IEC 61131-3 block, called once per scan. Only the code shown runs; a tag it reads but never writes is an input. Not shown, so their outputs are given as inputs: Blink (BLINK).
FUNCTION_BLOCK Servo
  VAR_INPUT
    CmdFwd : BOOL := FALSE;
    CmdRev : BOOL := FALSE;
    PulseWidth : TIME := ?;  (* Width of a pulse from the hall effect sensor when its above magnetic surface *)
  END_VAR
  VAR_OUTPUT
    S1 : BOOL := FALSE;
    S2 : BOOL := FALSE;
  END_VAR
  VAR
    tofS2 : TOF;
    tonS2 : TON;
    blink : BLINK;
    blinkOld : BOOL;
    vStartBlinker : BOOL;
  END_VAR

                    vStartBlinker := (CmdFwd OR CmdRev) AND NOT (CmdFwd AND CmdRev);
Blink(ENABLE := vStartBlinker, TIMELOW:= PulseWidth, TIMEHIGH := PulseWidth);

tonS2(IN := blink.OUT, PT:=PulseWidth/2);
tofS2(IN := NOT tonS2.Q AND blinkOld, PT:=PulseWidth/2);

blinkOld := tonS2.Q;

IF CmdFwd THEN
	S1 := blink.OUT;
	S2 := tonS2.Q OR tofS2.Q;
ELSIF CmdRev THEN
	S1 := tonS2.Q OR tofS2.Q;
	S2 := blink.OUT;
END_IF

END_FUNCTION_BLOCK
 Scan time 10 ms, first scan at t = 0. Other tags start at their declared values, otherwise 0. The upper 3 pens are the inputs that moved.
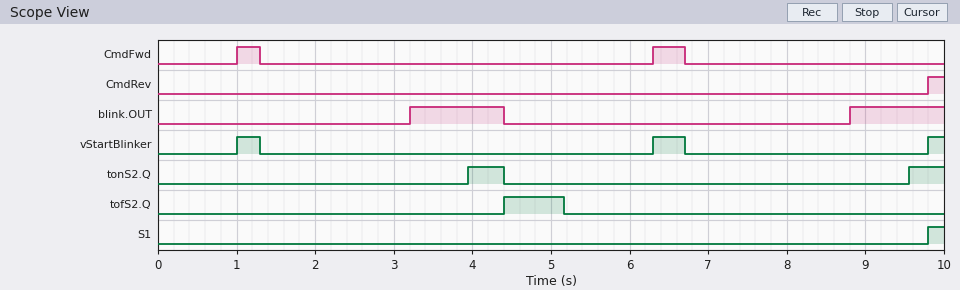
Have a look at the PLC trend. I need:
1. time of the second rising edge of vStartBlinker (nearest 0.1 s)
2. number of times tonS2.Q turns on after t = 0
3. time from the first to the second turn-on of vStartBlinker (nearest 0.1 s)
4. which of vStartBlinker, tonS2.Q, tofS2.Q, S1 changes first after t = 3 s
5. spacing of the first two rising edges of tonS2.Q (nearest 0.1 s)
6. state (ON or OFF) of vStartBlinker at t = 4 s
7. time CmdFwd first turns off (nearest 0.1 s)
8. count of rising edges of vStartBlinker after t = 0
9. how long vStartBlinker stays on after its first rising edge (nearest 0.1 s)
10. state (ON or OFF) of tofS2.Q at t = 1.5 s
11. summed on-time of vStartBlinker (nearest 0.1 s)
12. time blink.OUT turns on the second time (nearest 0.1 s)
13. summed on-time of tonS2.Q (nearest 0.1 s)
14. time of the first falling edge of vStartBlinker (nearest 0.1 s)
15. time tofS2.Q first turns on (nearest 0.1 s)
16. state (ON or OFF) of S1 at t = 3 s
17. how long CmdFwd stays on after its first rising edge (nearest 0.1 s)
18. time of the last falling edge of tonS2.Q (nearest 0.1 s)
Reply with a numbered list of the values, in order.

1. 6.3 s
2. 2
3. 5.3 s
4. tonS2.Q
5. 5.6 s
6. OFF
7. 1.3 s
8. 3
9. 0.3 s
10. OFF
11. 0.9 s
12. 8.8 s
13. 0.9 s
14. 1.3 s
15. 4.4 s
16. OFF
17. 0.3 s
18. 4.4 s
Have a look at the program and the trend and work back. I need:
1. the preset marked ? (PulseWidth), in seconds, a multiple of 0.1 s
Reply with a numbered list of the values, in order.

1. 1.5 s
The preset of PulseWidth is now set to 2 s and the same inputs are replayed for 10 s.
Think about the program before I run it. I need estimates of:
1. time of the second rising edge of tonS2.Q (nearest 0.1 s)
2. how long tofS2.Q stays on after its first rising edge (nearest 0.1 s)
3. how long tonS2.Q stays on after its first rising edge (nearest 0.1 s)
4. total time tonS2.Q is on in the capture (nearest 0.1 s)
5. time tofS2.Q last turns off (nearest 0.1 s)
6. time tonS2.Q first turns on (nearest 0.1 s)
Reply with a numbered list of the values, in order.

1. 9.8 s
2. 1.0 s
3. 0.2 s
4. 0.4 s
5. 5.4 s
6. 4.2 s
